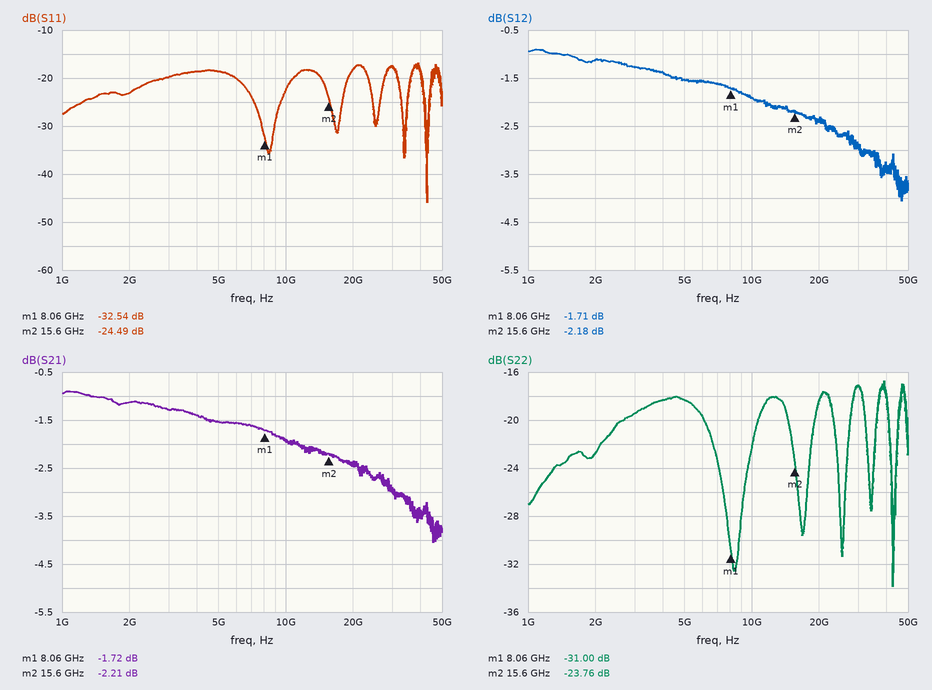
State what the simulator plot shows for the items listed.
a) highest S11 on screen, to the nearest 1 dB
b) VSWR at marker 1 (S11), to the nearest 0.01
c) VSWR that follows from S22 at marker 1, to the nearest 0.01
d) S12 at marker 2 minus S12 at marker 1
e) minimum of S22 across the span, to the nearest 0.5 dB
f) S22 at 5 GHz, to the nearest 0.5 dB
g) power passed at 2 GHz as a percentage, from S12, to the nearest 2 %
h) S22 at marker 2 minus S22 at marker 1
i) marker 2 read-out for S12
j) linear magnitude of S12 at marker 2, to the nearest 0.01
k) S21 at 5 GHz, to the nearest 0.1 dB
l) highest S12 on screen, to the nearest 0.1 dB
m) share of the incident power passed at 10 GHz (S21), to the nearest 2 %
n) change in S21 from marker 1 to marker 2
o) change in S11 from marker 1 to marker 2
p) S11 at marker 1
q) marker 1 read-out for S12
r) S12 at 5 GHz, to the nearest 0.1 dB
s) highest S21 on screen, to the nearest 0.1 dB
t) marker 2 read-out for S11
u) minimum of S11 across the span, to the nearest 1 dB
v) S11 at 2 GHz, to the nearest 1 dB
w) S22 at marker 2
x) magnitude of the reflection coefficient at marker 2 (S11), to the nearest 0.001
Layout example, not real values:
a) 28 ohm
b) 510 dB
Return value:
a) -17 dB
b) 1.05
c) 1.06
d) -0.47 dB
e) -34.0 dB
f) -18.5 dB
g) 78 %
h) 7.24 dB
i) -2.18 dB
j) 0.78
k) -1.5 dB
l) -0.9 dB
m) 64 %
n) -0.49 dB
o) 8.05 dB
p) -32.54 dB
q) -1.71 dB
r) -1.5 dB
s) -0.9 dB
t) -24.49 dB
u) -46 dB
v) -23 dB
w) -23.76 dB
x) 0.060
